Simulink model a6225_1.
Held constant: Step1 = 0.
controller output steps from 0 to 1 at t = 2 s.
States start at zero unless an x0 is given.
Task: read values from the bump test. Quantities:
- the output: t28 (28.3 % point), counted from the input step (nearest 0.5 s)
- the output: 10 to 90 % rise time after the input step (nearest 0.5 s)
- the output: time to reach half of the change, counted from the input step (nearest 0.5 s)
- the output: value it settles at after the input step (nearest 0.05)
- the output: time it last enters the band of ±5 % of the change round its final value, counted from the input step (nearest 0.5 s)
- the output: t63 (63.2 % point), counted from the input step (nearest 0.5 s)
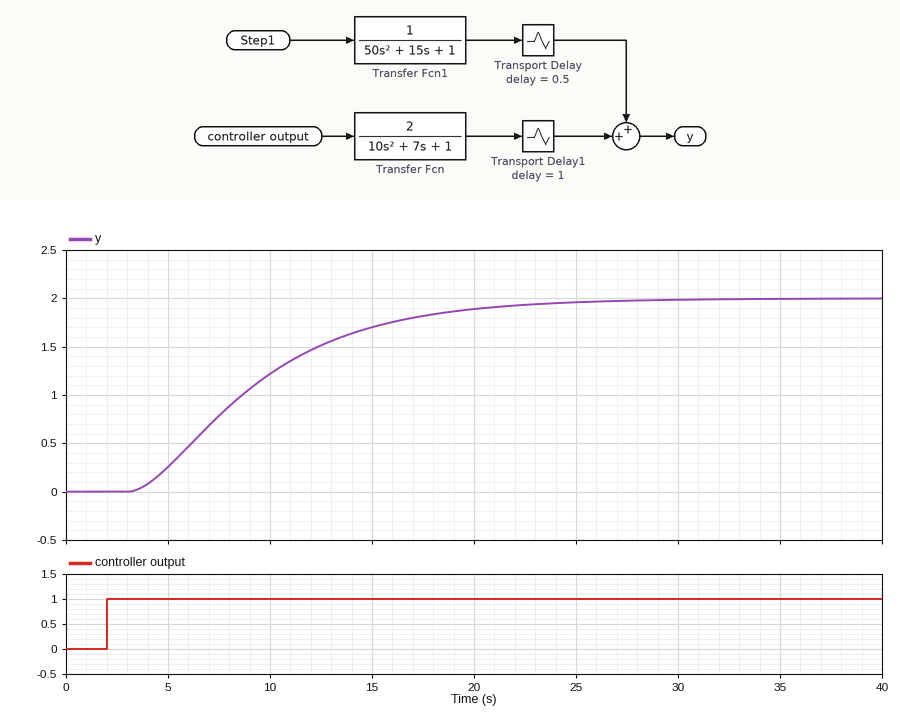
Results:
4.5 s
12.5 s
6.5 s
2.00
18.5 s
8.5 s
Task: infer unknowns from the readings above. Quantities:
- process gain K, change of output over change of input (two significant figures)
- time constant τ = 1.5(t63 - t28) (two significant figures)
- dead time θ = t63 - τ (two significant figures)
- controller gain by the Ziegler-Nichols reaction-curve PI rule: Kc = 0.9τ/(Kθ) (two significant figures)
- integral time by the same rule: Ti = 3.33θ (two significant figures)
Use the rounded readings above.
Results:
2.0
6.0 s
2.5 s
1.1
8.3 s
